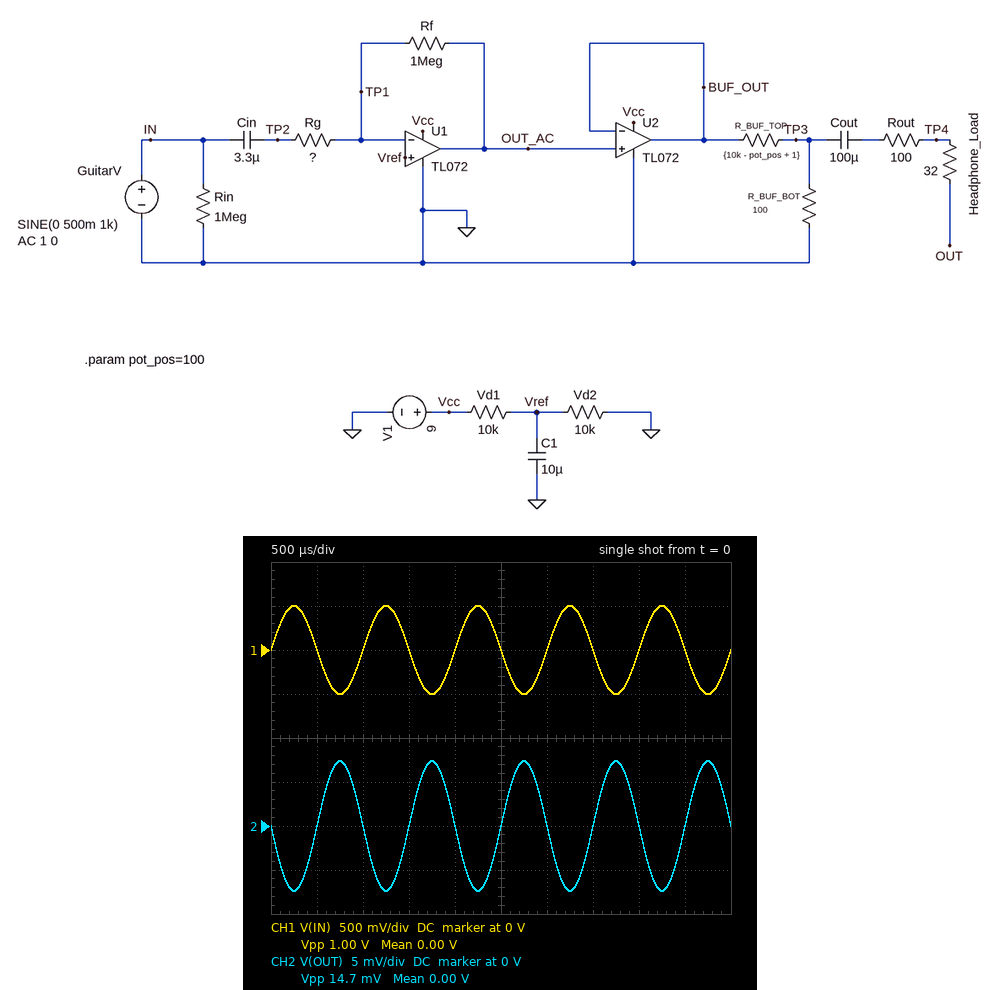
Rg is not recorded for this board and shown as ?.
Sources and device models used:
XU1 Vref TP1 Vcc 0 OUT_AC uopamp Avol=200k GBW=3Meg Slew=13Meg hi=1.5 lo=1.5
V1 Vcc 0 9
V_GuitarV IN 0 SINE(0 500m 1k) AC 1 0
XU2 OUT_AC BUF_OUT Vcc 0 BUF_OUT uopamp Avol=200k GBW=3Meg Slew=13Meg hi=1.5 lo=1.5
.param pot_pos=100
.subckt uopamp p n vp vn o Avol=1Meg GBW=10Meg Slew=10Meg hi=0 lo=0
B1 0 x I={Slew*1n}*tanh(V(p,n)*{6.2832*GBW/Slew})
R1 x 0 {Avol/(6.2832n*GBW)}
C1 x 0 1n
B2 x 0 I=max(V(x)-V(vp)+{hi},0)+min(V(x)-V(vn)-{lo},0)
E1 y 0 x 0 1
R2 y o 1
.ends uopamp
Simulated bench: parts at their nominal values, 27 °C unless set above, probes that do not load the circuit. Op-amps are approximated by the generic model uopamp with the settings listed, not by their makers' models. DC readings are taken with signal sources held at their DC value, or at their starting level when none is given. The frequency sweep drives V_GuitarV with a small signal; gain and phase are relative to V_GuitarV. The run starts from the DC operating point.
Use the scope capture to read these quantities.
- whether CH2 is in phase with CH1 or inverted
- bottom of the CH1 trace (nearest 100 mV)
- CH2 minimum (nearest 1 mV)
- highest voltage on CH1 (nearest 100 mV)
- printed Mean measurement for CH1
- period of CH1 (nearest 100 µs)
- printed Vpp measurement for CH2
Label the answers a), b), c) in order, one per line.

a) inverted
b) -500 mV
c) -7 mV
d) 500 mV
e) 0.00 V
f) 1.0 ms
g) 14.7 mV
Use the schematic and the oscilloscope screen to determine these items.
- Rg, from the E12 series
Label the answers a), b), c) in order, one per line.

a) 680 kΩ
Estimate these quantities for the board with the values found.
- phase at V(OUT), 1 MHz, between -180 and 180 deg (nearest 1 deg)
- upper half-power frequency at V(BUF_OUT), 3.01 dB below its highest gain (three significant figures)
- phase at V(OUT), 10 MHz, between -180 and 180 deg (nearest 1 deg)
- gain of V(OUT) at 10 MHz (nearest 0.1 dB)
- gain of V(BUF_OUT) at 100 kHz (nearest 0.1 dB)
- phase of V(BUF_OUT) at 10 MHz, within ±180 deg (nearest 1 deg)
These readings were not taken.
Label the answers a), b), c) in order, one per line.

a) 122 deg
b) 1.07 MHz
c) 24 deg
d) -65.9 dB
e) 3.3 dB
f) 24 deg
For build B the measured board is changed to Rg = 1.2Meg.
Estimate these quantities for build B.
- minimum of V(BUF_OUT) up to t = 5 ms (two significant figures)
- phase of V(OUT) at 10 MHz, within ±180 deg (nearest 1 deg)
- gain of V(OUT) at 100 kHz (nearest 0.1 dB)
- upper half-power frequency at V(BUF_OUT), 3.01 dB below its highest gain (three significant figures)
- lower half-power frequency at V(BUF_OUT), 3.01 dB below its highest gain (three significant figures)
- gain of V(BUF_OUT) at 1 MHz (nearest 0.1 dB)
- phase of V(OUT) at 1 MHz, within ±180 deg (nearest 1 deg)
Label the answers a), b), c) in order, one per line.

a) 4.1 V
b) 26 deg
c) -41.6 dB
d) 1.34 MHz
e) 40.2 mHz
f) -3.4 dB
g) 130 deg
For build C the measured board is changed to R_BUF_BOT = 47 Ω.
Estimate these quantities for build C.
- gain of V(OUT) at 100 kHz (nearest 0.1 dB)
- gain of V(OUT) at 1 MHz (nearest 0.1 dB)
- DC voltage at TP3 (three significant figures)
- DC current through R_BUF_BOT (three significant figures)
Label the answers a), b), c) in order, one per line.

a) -43.2 dB
b) -45.9 dB
c) 21.3 mV
d) 452 µA
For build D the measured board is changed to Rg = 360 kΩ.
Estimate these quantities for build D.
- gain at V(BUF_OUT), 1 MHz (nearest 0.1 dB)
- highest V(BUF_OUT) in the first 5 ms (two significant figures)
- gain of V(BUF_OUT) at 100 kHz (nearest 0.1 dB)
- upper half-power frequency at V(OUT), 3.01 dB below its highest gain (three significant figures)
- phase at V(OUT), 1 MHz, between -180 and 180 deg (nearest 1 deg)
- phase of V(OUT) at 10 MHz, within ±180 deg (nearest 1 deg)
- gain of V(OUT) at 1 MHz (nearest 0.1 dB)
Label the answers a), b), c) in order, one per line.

a) 4.3 dB
b) 5.9 V
c) 8.8 dB
d) 746 kHz
e) 110 deg
f) 21 deg
g) -35.7 dB
